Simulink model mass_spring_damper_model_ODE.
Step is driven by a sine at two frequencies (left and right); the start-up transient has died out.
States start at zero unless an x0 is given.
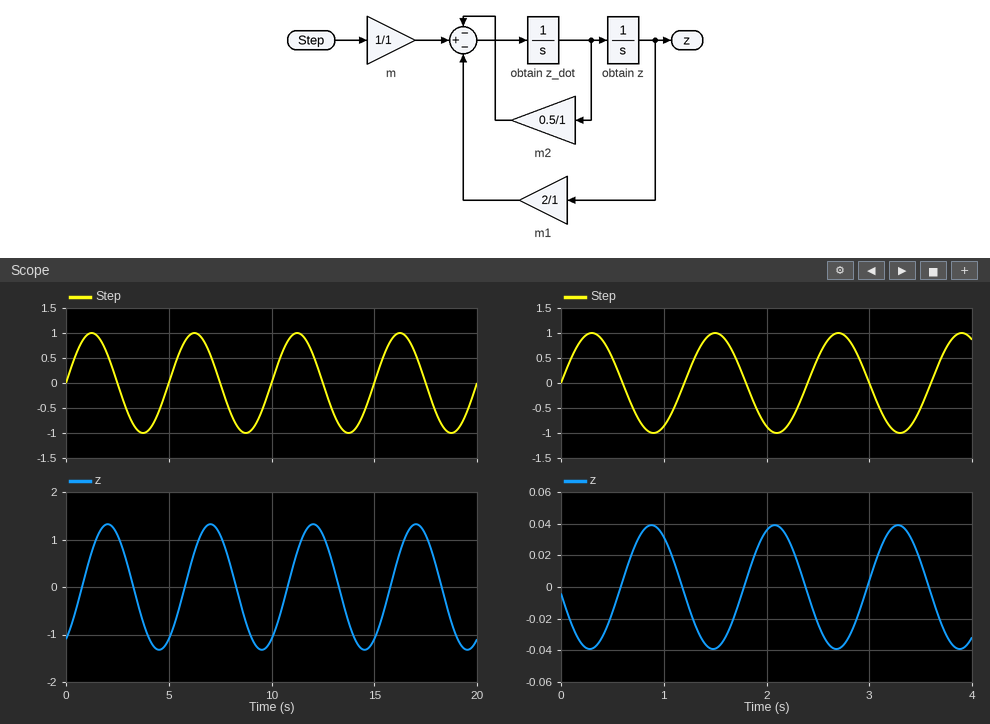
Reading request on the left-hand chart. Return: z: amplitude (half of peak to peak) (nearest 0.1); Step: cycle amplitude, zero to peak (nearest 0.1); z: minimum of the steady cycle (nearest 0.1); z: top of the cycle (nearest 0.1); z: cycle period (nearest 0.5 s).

1.3
1.0
-1.3
1.3
5.0 s
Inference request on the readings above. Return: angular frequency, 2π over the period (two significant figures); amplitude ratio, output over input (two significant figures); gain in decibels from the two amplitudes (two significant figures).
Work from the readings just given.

1.3 rad/s
1.3
2.3 dB
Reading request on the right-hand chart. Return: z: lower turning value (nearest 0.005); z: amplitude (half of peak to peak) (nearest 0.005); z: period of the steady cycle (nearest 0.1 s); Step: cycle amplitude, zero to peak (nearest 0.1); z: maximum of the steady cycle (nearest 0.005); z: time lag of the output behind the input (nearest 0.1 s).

-0.040
0.040
1.2 s
1.0
0.040
0.6 s
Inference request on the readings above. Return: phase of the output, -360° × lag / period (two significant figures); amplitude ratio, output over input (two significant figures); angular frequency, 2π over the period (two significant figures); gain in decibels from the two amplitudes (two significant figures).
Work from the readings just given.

-180°
0.040
5.2 rad/s
-28 dB
